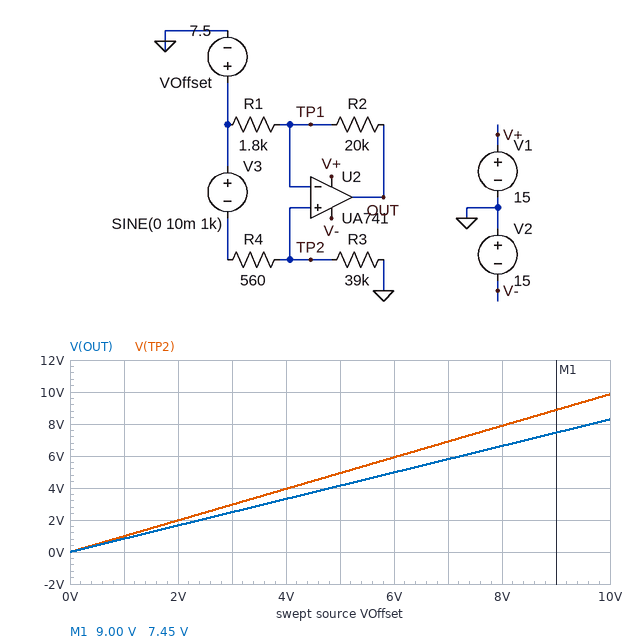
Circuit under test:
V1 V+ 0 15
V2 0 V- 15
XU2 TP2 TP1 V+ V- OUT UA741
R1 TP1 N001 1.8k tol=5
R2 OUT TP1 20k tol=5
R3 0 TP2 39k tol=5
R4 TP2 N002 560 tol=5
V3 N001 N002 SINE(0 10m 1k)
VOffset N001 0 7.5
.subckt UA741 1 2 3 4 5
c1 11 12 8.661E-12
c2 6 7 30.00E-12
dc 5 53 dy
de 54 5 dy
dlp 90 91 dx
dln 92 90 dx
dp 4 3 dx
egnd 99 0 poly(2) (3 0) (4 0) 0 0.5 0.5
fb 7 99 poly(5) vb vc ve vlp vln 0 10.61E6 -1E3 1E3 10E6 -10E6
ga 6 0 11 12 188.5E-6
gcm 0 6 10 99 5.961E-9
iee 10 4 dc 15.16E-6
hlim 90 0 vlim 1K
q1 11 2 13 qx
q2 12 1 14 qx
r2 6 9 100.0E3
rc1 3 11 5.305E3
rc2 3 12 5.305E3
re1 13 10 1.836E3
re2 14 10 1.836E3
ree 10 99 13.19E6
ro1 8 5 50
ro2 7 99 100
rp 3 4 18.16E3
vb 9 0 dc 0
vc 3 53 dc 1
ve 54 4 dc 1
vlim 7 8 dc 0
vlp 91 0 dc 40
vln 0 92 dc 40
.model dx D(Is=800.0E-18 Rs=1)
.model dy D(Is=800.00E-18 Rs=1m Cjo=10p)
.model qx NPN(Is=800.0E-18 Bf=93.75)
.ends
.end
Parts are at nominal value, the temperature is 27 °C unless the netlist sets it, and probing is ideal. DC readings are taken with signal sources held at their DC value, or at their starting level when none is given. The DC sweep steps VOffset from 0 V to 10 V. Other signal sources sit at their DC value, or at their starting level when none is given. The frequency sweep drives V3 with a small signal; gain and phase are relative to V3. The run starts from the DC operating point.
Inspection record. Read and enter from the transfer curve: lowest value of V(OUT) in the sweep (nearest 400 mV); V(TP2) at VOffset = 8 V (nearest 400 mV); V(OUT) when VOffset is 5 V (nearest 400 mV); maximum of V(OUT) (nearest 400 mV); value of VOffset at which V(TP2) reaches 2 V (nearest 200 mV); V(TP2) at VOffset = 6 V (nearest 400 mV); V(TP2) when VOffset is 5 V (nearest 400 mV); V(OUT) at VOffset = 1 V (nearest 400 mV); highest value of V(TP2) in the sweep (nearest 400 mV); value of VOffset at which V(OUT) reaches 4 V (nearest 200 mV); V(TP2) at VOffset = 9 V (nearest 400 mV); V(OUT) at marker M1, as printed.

0 V
8.0 V
4.0 V
8.4 V
2.0 V
6.0 V
4.8 V
800 mV
10.0 V
4.8 V
8.8 V
7.45 V
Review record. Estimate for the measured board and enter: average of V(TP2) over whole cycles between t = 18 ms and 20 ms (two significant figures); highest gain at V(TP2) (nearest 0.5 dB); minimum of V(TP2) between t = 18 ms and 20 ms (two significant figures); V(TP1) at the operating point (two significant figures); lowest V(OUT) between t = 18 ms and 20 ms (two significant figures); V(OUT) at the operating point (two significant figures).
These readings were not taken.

7.4 V
0 dB
7.4 V
7.4 V
6.1 V
6.2 V
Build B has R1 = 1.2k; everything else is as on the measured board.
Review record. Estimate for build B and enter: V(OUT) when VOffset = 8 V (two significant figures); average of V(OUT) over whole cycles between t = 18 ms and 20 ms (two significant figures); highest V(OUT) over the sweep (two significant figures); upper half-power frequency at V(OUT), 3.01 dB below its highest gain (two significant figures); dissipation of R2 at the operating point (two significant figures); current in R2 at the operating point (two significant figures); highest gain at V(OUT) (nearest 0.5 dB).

6.0 V
5.6 V
7.5 V
60 kHz
160 µW
89 µA
25.0 dB
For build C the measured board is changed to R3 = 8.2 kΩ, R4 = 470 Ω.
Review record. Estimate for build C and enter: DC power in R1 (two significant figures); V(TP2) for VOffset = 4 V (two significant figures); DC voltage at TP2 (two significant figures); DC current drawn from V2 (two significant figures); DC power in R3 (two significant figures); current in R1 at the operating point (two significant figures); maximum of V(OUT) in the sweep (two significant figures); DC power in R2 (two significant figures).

92 µW
3.8 V
7.1 V
1.7 mA
6.1 mW
230 µA
3.4 V
1.0 mW
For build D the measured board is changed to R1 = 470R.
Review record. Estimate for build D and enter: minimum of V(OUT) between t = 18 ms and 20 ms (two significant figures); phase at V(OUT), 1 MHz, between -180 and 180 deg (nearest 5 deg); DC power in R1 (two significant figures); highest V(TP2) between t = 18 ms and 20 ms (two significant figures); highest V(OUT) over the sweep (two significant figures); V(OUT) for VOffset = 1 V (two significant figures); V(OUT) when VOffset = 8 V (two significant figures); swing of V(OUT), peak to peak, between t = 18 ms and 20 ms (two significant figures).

2.4 V
60 deg
24 µW
7.4 V
3.8 V
380 mV
3.1 V
860 mV
